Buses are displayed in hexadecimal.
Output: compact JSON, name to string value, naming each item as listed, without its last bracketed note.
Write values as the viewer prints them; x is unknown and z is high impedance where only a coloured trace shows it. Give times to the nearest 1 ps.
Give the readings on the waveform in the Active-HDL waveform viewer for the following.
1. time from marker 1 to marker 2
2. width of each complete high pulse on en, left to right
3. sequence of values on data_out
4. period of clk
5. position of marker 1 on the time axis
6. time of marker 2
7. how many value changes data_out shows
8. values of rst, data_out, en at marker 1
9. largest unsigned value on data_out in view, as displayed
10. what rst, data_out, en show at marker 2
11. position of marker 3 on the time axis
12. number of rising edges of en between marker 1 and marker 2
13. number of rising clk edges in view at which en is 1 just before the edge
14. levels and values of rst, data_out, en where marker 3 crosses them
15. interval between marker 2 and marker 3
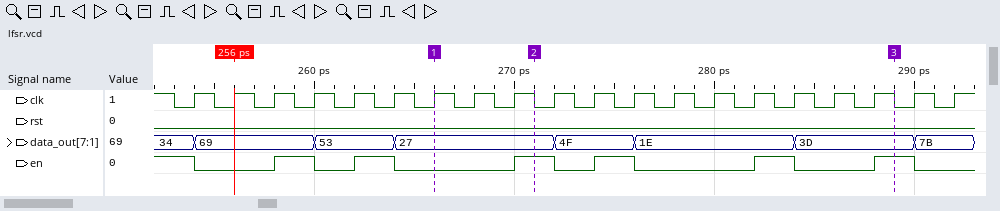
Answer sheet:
{"time from marker 1 to marker 2": "5 ps", "width of each complete high pulse on en, left to right": "2 ps, 2 ps, 2 ps, 2 ps, 2 ps, 2 ps", "sequence of values on data_out": "34, 69, 53, 27, 4F, 1E, 3D, 7B", "period of clk": "2 ps", "position of marker 1 on the time axis": "266 ps", "time of marker 2": "271 ps", "how many value changes data_out shows": "7", "values of rst, data_out, en at marker 1": "rst=0, data_out=27, en=0", "largest unsigned value on data_out in view, as displayed": "7B", "what rst, data_out, en show at marker 2": "rst=0, data_out=27, en=1", "position of marker 3 on the time axis": "289 ps", "number of rising edges of en between marker 1 and marker 2": "1", "number of rising clk edges in view at which en is 1 just before the edge": "7", "levels and values of rst, data_out, en where marker 3 crosses them": "rst=0, data_out=3D, en=1", "interval between marker 2 and marker 3": "18 ps"}
